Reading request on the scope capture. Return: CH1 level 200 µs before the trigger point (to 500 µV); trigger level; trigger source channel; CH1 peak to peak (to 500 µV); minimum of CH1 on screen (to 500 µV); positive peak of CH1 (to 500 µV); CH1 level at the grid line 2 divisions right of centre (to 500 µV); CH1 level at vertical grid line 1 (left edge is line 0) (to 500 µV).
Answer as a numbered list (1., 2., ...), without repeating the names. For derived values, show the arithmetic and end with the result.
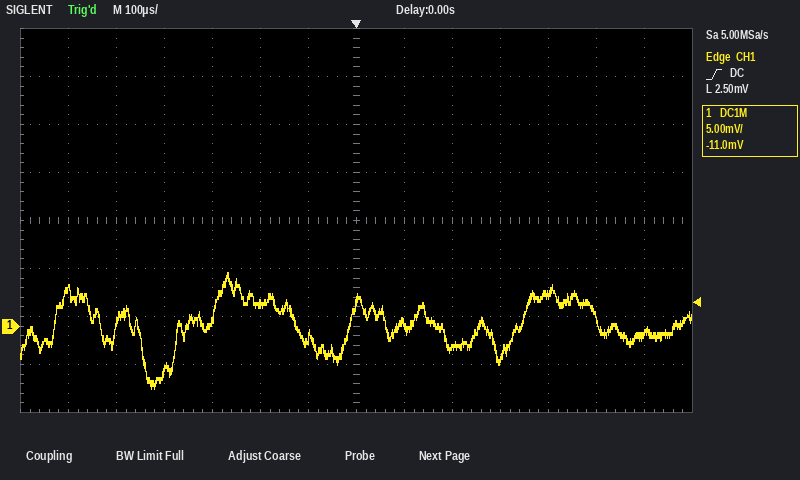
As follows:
1. 2.5 mV
2. 2.50 mV
3. CH1
4. 5.5 mV − (-6.5 mV) = 12.0 mV
5. -6.5 mV
6. 5.5 mV
7. -2.0 mV
8. 4.0 mV
